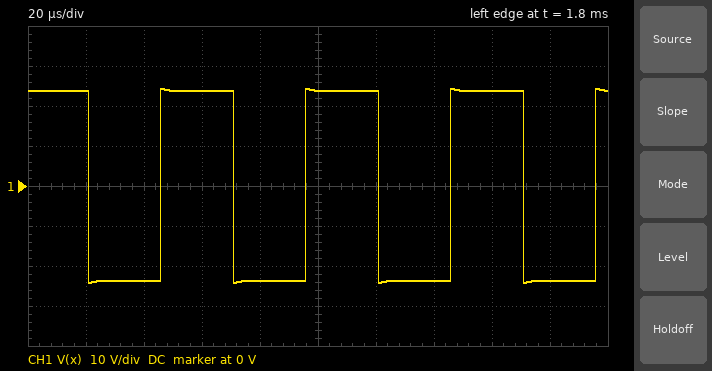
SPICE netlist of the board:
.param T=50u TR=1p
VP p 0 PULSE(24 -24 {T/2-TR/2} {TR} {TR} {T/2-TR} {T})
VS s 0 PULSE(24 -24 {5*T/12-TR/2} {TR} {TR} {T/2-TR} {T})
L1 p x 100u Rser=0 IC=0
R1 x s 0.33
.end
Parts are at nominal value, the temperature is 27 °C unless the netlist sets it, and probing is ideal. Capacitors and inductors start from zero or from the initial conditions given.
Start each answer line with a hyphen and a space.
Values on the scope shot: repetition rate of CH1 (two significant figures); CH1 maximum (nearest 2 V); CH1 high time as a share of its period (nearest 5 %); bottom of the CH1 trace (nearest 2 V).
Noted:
- 20 kHz
- 24 V
- 50 %
- -24 V
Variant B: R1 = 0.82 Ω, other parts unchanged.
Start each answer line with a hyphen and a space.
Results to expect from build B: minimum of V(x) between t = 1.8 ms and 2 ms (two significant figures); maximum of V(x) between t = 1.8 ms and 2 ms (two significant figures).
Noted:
- -25 V
- 25 V
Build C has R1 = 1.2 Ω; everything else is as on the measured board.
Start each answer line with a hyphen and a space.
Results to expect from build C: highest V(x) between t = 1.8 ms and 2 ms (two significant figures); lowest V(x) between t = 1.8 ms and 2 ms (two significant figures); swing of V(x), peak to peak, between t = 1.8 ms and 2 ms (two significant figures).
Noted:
- 25 V
- -25 V
- 50 V
